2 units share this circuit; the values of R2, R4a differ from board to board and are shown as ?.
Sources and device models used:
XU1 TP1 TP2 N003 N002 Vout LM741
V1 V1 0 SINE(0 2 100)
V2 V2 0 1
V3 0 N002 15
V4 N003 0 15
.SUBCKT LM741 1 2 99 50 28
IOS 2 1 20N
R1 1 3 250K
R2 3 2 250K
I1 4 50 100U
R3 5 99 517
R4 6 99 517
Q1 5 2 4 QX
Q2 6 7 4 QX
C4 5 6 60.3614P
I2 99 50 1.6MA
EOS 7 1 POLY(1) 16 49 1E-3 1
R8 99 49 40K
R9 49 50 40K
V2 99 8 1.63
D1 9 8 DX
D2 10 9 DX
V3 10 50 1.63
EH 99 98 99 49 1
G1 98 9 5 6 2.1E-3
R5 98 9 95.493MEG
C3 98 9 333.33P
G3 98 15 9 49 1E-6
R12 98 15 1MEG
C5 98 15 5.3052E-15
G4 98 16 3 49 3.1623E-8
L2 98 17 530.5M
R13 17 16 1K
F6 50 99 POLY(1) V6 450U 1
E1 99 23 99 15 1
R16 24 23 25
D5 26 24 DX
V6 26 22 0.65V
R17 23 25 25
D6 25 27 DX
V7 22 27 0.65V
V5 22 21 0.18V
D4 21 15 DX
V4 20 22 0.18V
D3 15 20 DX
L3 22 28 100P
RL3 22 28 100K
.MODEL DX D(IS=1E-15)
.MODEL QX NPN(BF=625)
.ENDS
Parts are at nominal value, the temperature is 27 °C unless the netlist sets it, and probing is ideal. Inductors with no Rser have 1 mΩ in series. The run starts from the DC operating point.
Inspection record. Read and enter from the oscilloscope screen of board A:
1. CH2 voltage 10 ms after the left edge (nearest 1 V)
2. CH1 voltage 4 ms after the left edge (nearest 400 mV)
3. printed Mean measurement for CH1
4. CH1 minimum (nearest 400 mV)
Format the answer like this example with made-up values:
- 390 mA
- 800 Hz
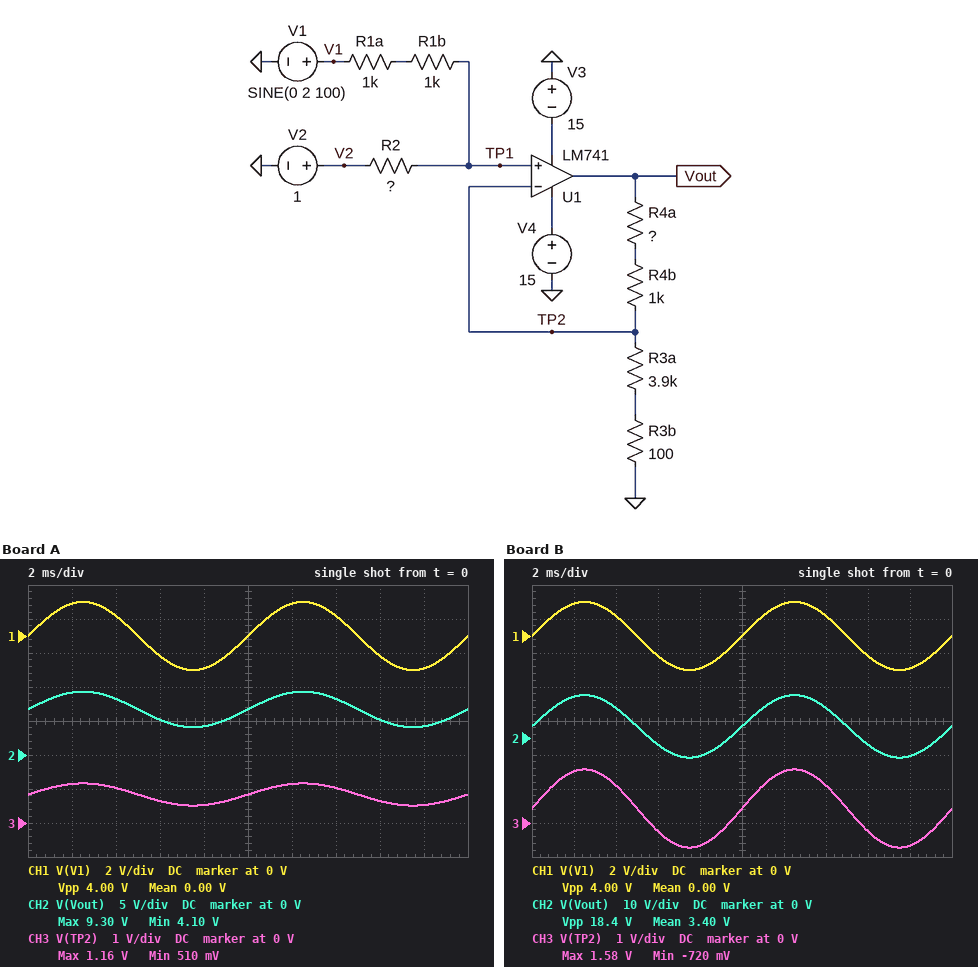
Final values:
- 7 V
- 1.2 V
- 0.00 V
- -2.0 V
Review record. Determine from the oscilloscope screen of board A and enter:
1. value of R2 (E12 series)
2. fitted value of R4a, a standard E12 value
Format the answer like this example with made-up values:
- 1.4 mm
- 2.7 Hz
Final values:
- 390 Ω
- 27 kΩ
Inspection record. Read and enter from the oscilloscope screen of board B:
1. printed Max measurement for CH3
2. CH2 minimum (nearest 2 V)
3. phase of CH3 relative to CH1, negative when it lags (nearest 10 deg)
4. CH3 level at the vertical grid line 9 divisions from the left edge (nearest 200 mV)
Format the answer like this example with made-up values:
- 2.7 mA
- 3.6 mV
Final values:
- 1.58 V
- -6 V
- 0 deg
- -600 mV
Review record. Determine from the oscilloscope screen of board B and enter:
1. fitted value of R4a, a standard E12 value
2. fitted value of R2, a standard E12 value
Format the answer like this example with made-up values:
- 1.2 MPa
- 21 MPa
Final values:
- 27 kΩ
- 2.7 kΩ
